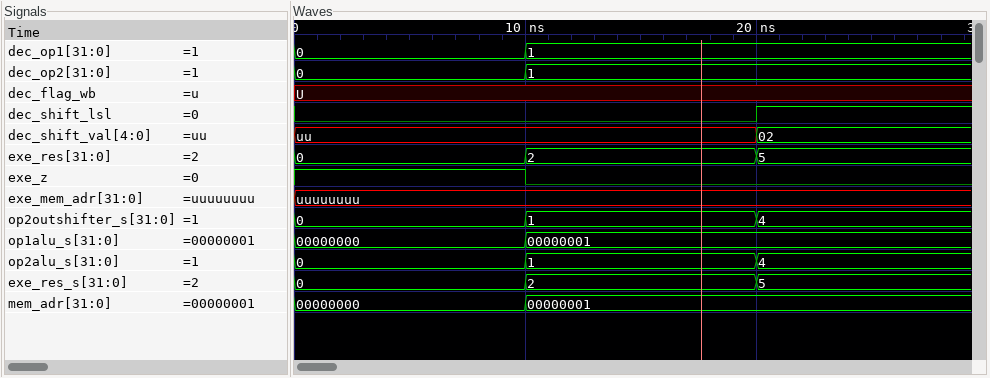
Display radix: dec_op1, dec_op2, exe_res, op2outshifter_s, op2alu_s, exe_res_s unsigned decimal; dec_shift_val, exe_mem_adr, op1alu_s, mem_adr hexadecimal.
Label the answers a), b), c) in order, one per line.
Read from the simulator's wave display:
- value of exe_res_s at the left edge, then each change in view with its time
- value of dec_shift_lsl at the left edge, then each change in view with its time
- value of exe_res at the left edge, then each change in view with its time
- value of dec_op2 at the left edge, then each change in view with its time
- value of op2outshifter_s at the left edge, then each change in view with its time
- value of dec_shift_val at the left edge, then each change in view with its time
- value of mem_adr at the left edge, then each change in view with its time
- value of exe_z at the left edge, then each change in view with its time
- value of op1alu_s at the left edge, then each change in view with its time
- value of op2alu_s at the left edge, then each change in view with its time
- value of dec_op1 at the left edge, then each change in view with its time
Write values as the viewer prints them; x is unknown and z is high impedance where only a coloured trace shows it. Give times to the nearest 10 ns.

a) 0, 2 at 10 ns, 5 at 20 ns
b) 0, 1 at 20 ns
c) 0, 2 at 10 ns, 5 at 20 ns
d) 0, 1 at 10 ns
e) 0, 1 at 10 ns, 4 at 20 ns
f) uu, 02 at 20 ns
g) 00000000, 00000001 at 10 ns
h) 1, 0 at 10 ns
i) 00000000, 00000001 at 10 ns
j) 0, 1 at 10 ns, 4 at 20 ns
k) 0, 1 at 10 ns
